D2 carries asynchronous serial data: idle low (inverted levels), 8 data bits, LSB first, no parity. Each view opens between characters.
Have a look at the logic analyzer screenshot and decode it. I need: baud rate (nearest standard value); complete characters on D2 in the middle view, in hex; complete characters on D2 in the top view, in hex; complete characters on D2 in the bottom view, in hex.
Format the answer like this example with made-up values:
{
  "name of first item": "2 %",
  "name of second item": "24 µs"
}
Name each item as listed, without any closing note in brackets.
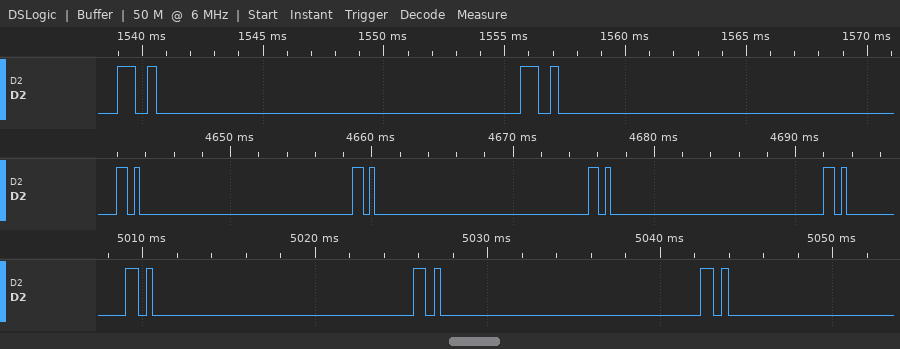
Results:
{
  "baud rate": "2400 baud",
  "complete characters on D2 in the middle view, in hex": "FA, FA, FA, FA",
  "complete characters on D2 in the top view, in hex": "FA, FA",
  "complete characters on D2 in the bottom view, in hex": "FA, FA, FA"
}
